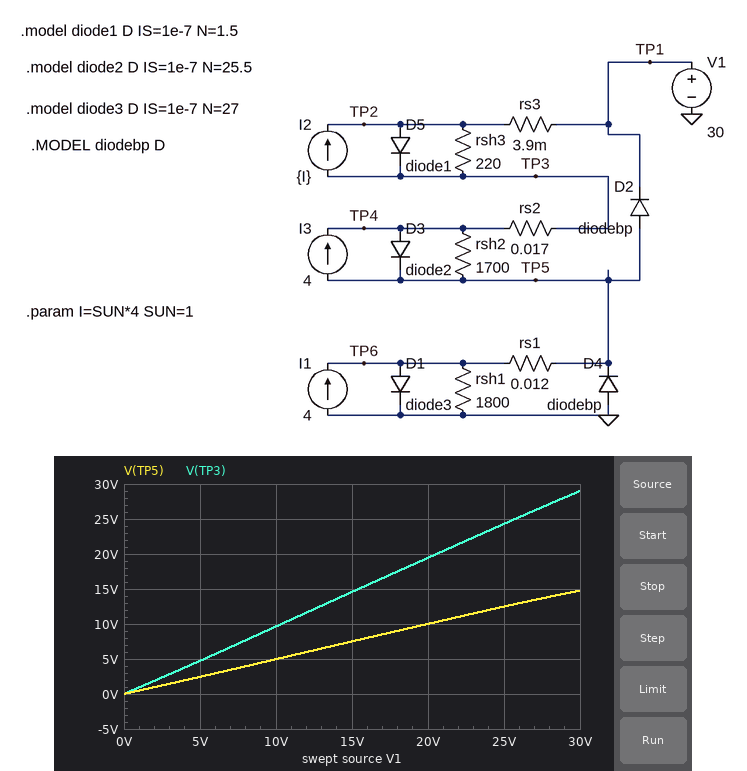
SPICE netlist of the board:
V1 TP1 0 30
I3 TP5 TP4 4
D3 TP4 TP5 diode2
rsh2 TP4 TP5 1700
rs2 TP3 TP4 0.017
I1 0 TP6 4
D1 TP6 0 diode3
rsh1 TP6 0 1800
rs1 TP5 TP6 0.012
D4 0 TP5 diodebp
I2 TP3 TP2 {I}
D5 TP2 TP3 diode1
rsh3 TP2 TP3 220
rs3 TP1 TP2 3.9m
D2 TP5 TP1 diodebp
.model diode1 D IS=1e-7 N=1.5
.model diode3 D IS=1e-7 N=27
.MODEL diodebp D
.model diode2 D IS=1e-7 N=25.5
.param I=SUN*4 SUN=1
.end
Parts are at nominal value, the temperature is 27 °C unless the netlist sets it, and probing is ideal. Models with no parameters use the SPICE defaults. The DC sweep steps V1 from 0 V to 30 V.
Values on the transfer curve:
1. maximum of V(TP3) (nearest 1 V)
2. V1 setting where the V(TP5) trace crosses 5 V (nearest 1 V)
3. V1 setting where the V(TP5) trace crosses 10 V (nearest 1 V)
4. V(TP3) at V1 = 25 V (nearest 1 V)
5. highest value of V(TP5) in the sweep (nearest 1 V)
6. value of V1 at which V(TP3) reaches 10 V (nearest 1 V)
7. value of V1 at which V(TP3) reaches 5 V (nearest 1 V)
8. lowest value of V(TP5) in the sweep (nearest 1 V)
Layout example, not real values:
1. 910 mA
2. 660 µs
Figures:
1. 29 V
2. 10 V
3. 20 V
4. 24 V
5. 15 V
6. 10 V
7. 5 V
8. 0 V
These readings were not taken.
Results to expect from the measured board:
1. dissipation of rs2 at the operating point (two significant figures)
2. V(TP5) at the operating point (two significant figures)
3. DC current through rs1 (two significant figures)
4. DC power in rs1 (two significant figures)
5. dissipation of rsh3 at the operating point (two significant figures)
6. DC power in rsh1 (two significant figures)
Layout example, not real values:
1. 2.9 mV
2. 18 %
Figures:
1. 51 W
2. 15 V
3. 55 A
4. 36 W
5. 2.8 mW
6. 110 mW
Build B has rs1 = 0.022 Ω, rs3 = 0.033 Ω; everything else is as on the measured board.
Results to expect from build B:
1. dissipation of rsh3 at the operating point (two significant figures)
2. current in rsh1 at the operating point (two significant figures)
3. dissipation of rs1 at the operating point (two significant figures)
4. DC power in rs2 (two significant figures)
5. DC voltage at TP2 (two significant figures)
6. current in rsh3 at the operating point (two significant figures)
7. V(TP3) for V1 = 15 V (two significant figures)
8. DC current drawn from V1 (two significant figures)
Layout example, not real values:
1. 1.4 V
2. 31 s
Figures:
1. 2.7 mW
2. 7.7 mA
3. 25 W
4. 19 W
5. 29 V
6. 3.5 mA
7. 15 V
8. 34 A
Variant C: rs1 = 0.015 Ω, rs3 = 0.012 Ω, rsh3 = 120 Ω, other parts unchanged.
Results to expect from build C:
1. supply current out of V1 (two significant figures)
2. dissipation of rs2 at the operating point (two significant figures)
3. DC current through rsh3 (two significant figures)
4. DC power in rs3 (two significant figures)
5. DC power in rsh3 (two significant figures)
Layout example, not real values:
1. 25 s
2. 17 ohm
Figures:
1. 46 A
2. 36 W
3. 6.5 mA
4. 25 W
5. 5.0 mW
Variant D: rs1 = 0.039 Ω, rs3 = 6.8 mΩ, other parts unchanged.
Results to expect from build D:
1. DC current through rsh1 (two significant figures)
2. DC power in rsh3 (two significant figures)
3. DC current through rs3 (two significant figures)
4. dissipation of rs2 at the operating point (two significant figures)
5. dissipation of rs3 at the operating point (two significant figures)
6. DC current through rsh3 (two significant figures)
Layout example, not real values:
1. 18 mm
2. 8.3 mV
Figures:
1. 7.7 mA
2. 2.7 mW
3. 37 A
4. 23 W
5. 9.2 W
6. 3.5 mA
